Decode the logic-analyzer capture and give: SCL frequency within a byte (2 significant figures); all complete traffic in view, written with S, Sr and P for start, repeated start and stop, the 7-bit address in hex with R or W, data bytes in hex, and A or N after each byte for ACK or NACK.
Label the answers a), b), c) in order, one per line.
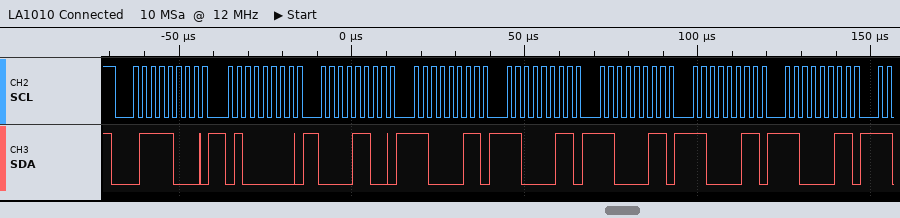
a) 400 kHz
b) S 3CW A 40 A 0C A C3 A C3 A C3 A C3 A C3 A
